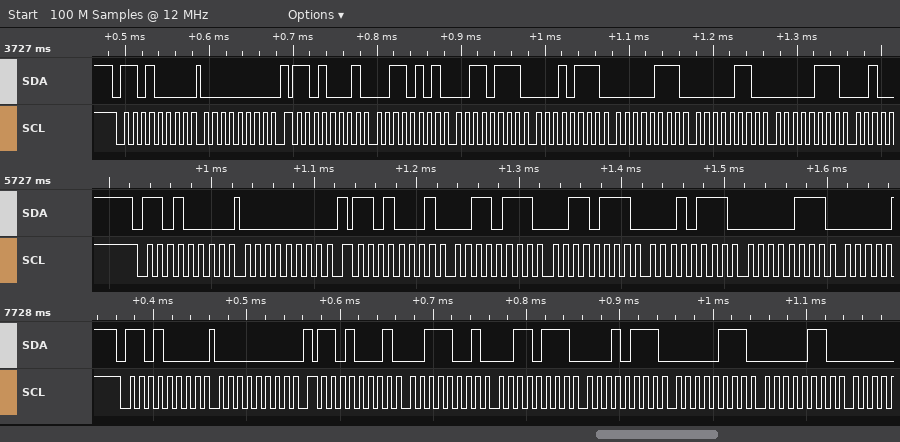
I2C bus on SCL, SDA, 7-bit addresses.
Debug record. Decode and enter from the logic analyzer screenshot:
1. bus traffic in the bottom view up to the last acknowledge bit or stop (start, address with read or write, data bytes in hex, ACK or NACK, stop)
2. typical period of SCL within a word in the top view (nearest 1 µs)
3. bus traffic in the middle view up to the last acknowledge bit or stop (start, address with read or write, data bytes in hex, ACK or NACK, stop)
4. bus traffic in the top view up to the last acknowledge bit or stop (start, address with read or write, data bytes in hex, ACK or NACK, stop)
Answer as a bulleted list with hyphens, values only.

- start, address 68 write ACK, 00 ACK, repeated start, address 68 read ACK, 39 ACK, 37 ACK, 17 ACK, 07 ACK, 06 ACK
- 10 µs
- start, address 68 write ACK, 00 ACK, repeated start, address 68 read ACK, 37 ACK, 37 ACK, 17 ACK, 07 ACK
- start, address 68 write ACK, 00 ACK, repeated start, address 68 read ACK, 35 ACK, 37 ACK, 17 ACK, 07 ACK, 06 ACK, 07 ACK
